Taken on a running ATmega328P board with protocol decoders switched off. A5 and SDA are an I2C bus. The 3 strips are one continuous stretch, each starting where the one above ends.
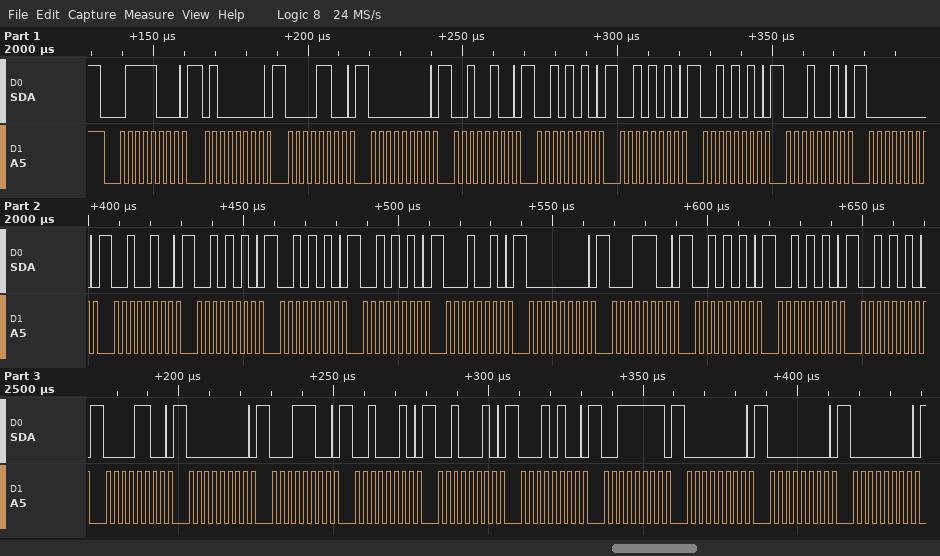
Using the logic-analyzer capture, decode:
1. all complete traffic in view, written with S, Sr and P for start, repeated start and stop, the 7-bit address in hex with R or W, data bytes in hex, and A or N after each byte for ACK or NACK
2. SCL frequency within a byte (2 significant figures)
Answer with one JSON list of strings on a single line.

["S 3CW A 40 A 0C A 00 A 24 A 2A A 2A A 2A A 12 A 00 A 24 A 2A A 2A A 2A A 12 A 00 A 1C A 2A A 2A A 2A A 0C A 00 A 1C A 22 A 22 A 14 A 3F A 00 A 00 A 00 A", "400 kHz"]
